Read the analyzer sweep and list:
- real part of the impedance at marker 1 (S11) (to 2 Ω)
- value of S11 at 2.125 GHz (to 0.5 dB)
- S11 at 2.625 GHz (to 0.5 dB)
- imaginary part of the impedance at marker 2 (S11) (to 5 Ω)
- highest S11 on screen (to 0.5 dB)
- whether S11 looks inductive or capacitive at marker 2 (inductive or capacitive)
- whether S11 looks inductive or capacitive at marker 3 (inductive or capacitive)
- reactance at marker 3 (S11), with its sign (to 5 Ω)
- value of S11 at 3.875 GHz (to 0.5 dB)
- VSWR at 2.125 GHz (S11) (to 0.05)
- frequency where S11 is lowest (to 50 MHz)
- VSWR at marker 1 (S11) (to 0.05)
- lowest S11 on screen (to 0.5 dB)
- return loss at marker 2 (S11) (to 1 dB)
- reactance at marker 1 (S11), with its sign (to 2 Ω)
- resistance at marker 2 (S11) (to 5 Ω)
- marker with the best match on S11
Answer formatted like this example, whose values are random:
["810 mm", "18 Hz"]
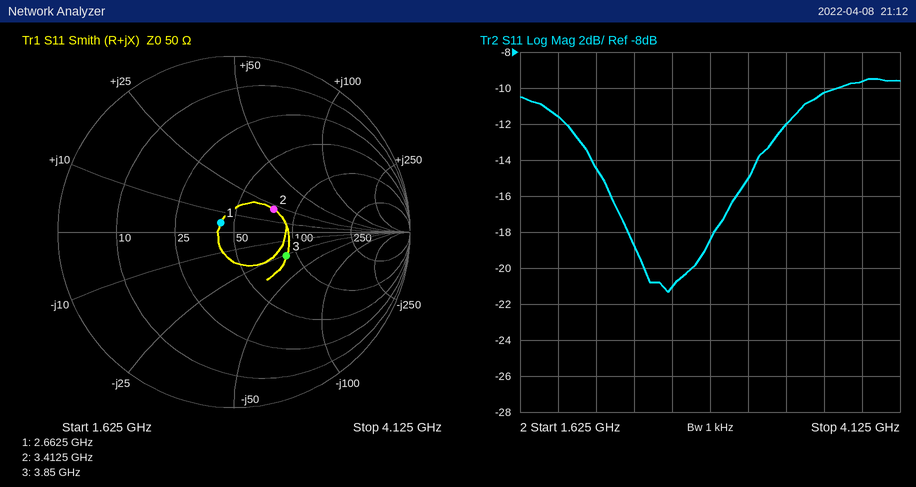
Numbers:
["42 Ω", "-14.5 dB", "-21.0 dB", "+20 Ω", "-9.5 dB", "inductive", "capacitive", "-25 Ω", "-9.5 dB", "1.45", "2.60 GHz", "1.20", "-21.5 dB", "12 dB", "+4 Ω", "75 Ω", "marker 1"]
